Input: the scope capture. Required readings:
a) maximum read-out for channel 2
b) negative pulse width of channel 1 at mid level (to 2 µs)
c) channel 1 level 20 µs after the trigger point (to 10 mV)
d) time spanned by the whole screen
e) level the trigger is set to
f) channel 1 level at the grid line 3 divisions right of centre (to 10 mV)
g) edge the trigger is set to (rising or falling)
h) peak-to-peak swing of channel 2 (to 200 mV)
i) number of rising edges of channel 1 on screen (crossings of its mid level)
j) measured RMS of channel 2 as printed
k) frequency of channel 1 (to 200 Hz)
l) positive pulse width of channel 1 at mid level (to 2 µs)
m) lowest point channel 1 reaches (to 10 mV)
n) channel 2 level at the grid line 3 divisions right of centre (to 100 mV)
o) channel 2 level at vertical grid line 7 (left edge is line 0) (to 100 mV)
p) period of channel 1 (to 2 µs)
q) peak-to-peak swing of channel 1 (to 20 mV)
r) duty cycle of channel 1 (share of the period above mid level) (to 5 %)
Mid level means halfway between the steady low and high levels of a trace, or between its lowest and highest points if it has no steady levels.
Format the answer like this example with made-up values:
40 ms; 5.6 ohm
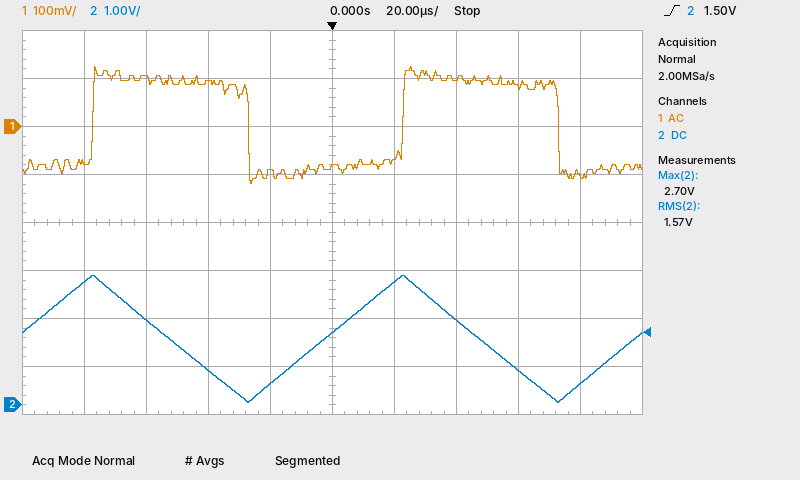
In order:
2.70 V; 50 µs; -70 mV; 200 µs; 1.50 V; 80 mV; rising; 2.6 V; 2; 1.57 V; 10.0 kHz; 50 µs; -120 mV; 700 mV; 1.8 V; 100 µs; 240 mV; 50 %
